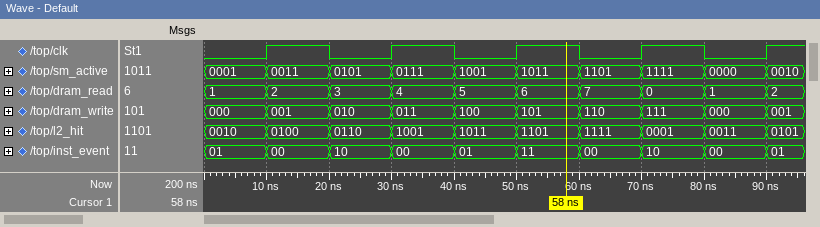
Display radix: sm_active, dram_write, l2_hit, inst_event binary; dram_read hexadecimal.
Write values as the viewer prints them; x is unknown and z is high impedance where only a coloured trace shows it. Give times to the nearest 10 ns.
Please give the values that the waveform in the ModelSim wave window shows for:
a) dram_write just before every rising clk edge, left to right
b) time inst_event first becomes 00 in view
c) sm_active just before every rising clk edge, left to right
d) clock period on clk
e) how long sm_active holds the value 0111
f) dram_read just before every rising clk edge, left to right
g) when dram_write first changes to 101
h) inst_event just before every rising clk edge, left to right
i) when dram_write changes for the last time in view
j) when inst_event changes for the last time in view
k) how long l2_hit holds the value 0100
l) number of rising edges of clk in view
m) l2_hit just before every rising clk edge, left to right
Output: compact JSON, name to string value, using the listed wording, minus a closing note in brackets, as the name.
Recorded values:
{"dram_write just before every rising clk edge, left to right": "000, 010, 100, 110, 000", "time inst_event first becomes 00 in view": "10 ns", "sm_active just before every rising clk edge, left to right": "0001, 0101, 1001, 1101, 0000", "clock period on clk": "20 ns", "how long sm_active holds the value 0111": "10 ns", "dram_read just before every rising clk edge, left to right": "1, 3, 5, 7, 1", "when dram_write first changes to 101": "50 ns", "inst_event just before every rising clk edge, left to right": "01, 10, 01, 00, 00", "when dram_write changes for the last time in view": "90 ns", "when inst_event changes for the last time in view": "90 ns", "how long l2_hit holds the value 0100": "10 ns", "number of rising edges of clk in view": "5", "l2_hit just before every rising clk edge, left to right": "0010, 0110, 1011, 1111, 0011"}
